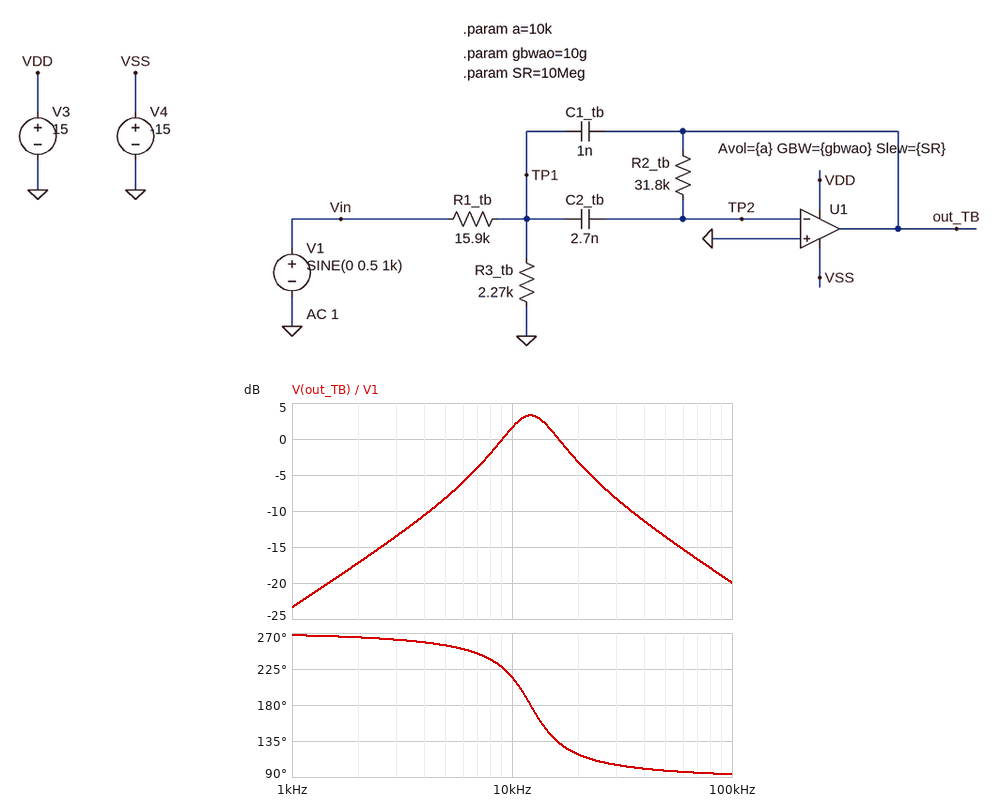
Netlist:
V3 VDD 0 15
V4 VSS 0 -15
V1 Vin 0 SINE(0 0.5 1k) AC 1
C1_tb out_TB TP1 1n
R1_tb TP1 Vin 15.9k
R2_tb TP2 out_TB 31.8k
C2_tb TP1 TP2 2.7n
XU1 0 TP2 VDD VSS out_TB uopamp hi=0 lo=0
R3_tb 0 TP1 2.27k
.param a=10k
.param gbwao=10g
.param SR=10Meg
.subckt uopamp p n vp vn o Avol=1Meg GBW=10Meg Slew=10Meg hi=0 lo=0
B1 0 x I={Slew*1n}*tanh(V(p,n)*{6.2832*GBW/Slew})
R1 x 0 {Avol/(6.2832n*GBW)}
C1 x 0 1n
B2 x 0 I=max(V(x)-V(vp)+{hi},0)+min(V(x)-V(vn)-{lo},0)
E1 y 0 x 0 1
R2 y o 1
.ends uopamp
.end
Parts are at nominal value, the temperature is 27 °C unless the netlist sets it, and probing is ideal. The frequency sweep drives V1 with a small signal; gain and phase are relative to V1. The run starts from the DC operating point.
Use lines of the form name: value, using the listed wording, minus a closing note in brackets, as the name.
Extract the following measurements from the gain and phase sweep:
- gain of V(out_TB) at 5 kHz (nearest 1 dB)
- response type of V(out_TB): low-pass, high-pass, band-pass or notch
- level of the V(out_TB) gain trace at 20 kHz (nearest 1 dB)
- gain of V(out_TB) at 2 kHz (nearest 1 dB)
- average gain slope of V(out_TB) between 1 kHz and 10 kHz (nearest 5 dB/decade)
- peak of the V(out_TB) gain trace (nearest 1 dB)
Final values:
gain of V(out_TB) at 5 kHz: -8 dB
response type of V(out_TB): low-pass, high-pass, band-pass or notch: band-pass
level of the V(out_TB) gain trace at 20 kHz: -3 dB
gain of V(out_TB) at 2 kHz: -17 dB
average gain slope of V(out_TB) between 1 kHz and 10 kHz: 25 dB/decade
peak of the V(out_TB) gain trace: 3 dB
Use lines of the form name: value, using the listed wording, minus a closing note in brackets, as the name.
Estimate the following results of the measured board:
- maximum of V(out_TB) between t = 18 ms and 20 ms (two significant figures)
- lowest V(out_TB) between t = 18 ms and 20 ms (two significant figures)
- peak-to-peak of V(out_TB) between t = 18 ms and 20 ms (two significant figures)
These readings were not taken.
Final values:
maximum of V(out_TB) between t = 18 ms and 20 ms: 34 mV
lowest V(out_TB) between t = 18 ms and 20 ms: -34 mV
peak-to-peak of V(out_TB) between t = 18 ms and 20 ms: 68 mV
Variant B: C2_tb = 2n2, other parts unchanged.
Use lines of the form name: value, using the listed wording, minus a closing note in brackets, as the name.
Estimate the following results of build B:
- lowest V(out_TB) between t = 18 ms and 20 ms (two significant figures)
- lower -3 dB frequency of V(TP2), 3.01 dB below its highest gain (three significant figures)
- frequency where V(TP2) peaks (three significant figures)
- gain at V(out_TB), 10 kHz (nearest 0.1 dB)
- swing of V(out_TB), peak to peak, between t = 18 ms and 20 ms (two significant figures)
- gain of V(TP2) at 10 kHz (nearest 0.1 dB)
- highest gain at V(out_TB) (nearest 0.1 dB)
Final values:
lowest V(out_TB) between t = 18 ms and 20 ms: -28 mV
lower -3 dB frequency of V(TP2), 3.01 dB below its highest gain: 11.5 kHz
frequency where V(TP2) peaks: 14.5 kHz
gain at V(out_TB), 10 kHz: -0.8 dB
swing of V(out_TB), peak to peak, between t = 18 ms and 20 ms: 55 mV
gain of V(TP2) at 10 kHz: -60.8 dB
highest gain at V(out_TB): 2.8 dB
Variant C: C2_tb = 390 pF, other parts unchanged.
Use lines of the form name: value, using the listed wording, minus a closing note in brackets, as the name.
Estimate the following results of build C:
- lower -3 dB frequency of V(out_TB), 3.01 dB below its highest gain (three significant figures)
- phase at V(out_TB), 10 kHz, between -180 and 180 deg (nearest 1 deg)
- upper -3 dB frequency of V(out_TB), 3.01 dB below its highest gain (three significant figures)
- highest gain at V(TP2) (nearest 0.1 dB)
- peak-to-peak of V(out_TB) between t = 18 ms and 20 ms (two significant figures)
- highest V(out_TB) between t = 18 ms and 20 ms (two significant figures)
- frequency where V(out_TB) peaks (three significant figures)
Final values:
lower -3 dB frequency of V(out_TB), 3.01 dB below its highest gain: 24.3 kHz
phase at V(out_TB), 10 kHz, between -180 and 180 deg: -101 deg
upper -3 dB frequency of V(out_TB), 3.01 dB below its highest gain: 42.0 kHz
highest gain at V(TP2): -54.6 dB
peak-to-peak of V(out_TB) between t = 18 ms and 20 ms: 9.7 mV
highest V(out_TB) between t = 18 ms and 20 ms: 4.9 mV
frequency where V(out_TB) peaks: 31.9 kHz
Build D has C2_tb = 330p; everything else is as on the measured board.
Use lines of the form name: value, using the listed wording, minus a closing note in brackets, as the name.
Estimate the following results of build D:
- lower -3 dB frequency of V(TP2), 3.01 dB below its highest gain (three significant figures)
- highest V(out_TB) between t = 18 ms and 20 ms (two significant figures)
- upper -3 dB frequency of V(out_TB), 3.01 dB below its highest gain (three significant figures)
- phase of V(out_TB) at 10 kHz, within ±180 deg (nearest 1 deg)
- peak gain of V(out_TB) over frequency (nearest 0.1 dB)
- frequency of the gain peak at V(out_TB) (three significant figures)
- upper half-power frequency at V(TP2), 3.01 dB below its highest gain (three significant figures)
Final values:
lower -3 dB frequency of V(TP2), 3.01 dB below its highest gain: 29.5 kHz
highest V(out_TB) between t = 18 ms and 20 ms: 4.1 mV
upper -3 dB frequency of V(out_TB), 3.01 dB below its highest gain: 46.1 kHz
phase of V(out_TB) at 10 kHz, within ±180 deg: -100 deg
peak gain of V(out_TB) over frequency: -6.1 dB
frequency of the gain peak at V(out_TB): 34.7 kHz
upper half-power frequency at V(TP2), 3.01 dB below its highest gain: 65.4 kHz
